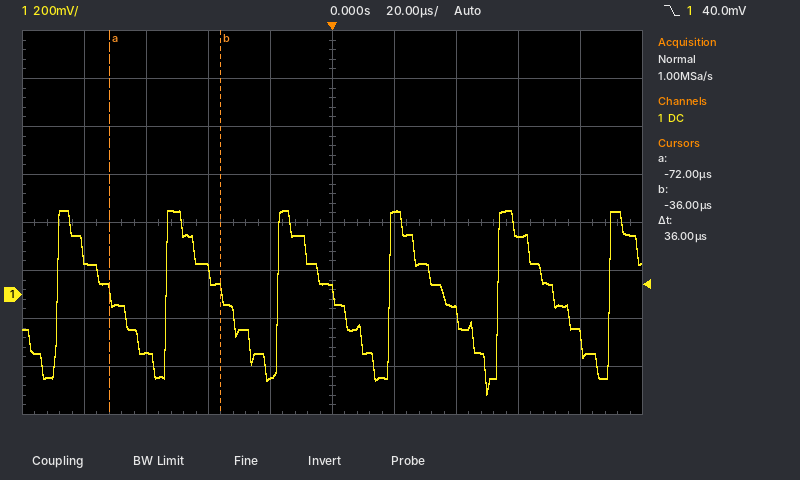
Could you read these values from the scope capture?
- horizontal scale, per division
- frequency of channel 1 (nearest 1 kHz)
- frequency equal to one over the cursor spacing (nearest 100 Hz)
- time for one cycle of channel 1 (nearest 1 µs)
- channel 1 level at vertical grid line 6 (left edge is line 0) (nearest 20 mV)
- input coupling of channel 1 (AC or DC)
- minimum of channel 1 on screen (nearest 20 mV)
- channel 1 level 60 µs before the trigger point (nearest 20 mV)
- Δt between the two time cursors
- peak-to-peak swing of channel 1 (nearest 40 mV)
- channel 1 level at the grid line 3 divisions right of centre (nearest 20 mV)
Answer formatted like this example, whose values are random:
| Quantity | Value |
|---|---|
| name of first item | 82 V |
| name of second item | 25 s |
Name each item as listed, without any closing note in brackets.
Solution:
| Quantity | Value |
|---|---|
| horizontal scale, per division | 20 µs |
| frequency of channel 1 | 28 kHz |
| frequency equal to one over the cursor spacing | 27.8 kHz |
| time for one cycle of channel 1 | 36 µs |
| channel 1 level at vertical grid line 6 (left edge is line 0) | 340 mV |
| input coupling of channel 1 | DC |
| minimum of channel 1 on screen | -420 mV |
| channel 1 level 60 µs before the trigger point | -240 mV |
| Δt between the two time cursors | 36 µs |
| peak-to-peak swing of channel 1 | 760 mV |
| channel 1 level at the grid line 3 divisions right of centre | 240 mV |
